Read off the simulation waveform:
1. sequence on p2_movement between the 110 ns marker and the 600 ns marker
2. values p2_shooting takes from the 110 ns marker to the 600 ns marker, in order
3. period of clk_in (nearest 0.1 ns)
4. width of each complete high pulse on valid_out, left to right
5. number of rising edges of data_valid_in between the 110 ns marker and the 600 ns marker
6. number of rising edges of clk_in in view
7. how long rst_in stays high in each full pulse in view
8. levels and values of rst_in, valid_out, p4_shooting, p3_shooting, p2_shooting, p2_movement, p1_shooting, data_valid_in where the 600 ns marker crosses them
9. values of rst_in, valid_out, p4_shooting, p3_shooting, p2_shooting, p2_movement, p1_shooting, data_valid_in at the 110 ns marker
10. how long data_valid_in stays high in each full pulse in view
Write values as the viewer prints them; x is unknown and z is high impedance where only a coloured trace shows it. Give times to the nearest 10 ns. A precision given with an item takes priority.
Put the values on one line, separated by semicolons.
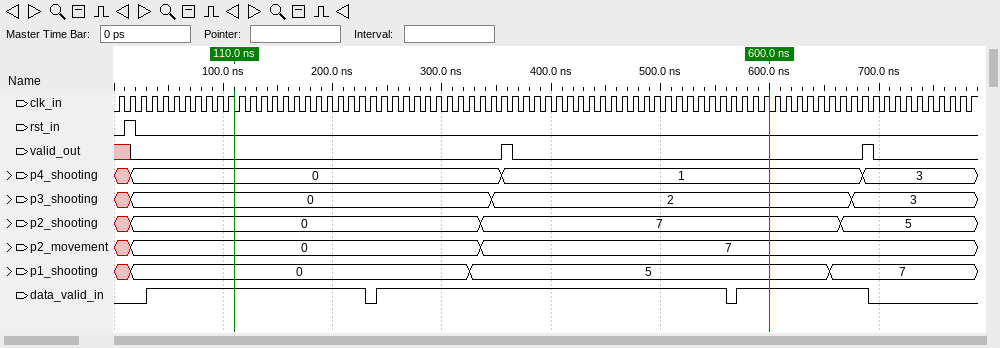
0, 7; 0, 7; 10 ns; 10 ns, 10 ns; 2; 79; 10 ns; rst_in=0, valid_out=0, p4_shooting=1, p3_shooting=2, p2_shooting=7, p2_movement=7, p1_shooting=5, data_valid_in=1; rst_in=0, valid_out=0, p4_shooting=0, p3_shooting=0, p2_shooting=0, p2_movement=0, p1_shooting=0, data_valid_in=1; 200 ns, 320 ns, 120 ns
